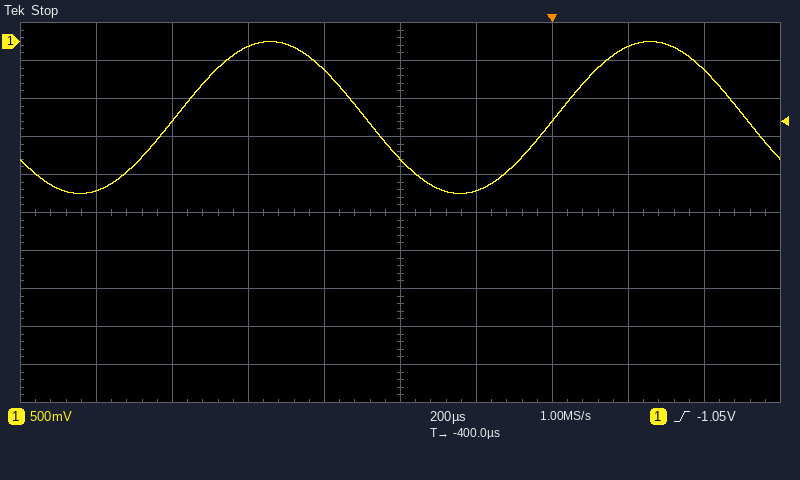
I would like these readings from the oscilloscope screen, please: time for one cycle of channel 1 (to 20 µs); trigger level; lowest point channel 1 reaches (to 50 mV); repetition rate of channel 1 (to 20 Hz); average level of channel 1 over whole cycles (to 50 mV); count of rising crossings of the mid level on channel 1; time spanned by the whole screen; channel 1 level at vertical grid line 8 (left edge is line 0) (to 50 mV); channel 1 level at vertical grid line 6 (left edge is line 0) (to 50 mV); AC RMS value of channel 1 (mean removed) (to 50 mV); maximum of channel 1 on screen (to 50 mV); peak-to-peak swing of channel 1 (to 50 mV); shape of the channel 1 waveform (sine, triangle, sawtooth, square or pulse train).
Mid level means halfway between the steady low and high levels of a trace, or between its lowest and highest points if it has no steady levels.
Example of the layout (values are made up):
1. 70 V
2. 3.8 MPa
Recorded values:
1. 1.00 ms
2. -1.05 V
3. -2.00 V
4. 1.00 kHz
5. -1.00 V
6. 2
7. 2 ms
8. -50 mV
9. -1.95 V
10. 700 mV
11. 0 mV
12. 2.00 V
13. sine
